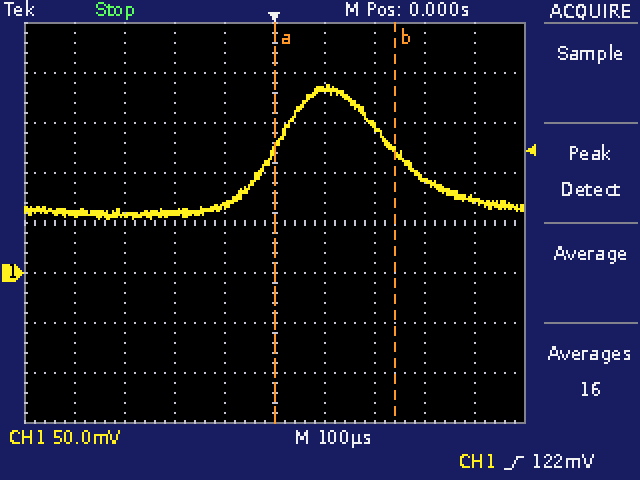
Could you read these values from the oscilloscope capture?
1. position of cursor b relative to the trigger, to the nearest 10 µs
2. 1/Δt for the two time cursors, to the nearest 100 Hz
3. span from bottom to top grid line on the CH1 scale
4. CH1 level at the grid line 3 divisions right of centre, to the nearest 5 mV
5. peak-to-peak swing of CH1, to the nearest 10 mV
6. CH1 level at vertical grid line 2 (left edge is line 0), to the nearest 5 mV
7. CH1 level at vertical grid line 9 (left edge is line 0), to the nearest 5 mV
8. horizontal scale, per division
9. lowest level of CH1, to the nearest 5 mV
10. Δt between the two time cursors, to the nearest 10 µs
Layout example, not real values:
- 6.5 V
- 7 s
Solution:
- +240 µs
- 4.2 kHz
- 400 mV
- 95 mV
- 130 mV
- 60 mV
- 75 mV
- 100 µs
- 55 mV
- 240 µs
